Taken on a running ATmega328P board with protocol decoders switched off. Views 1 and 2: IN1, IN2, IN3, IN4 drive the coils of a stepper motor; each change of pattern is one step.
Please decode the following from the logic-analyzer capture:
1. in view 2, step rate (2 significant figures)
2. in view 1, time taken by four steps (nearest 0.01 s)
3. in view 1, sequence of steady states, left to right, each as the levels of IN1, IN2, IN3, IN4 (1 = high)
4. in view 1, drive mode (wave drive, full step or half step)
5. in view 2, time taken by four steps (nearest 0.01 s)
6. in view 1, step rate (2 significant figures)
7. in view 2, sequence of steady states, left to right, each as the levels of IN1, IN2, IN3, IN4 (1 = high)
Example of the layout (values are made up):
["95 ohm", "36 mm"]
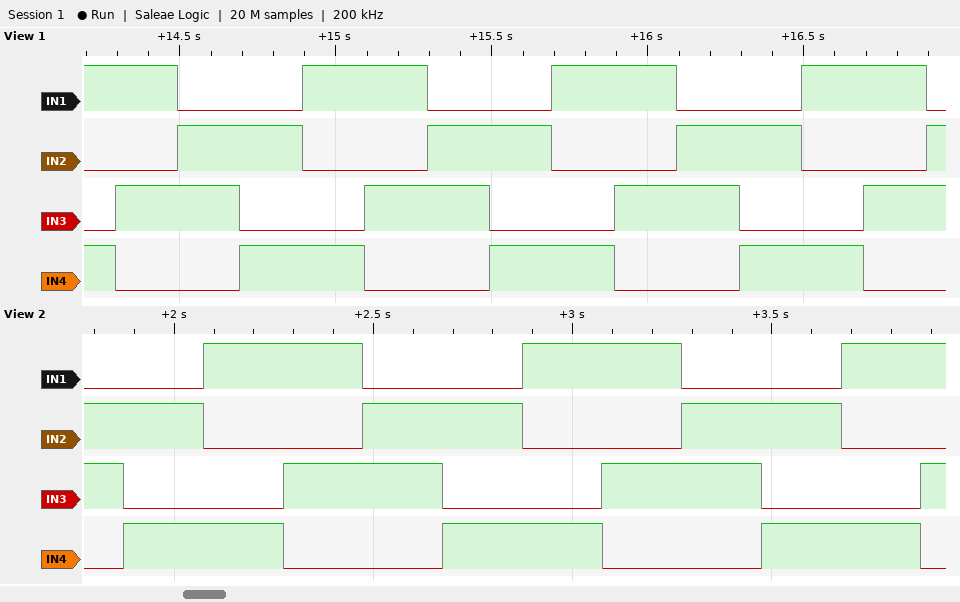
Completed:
["5.0 steps/s", "0.80 s", "1001 1010 0110 0101 1001 1010 0110 0101 1001 1010 0110 0101 1001 1010 0110", "full step", "0.80 s", "5.0 steps/s", "0110 0101 1001 1010 0110 0101 1001 1010 0110 0101 1001 1010"]
